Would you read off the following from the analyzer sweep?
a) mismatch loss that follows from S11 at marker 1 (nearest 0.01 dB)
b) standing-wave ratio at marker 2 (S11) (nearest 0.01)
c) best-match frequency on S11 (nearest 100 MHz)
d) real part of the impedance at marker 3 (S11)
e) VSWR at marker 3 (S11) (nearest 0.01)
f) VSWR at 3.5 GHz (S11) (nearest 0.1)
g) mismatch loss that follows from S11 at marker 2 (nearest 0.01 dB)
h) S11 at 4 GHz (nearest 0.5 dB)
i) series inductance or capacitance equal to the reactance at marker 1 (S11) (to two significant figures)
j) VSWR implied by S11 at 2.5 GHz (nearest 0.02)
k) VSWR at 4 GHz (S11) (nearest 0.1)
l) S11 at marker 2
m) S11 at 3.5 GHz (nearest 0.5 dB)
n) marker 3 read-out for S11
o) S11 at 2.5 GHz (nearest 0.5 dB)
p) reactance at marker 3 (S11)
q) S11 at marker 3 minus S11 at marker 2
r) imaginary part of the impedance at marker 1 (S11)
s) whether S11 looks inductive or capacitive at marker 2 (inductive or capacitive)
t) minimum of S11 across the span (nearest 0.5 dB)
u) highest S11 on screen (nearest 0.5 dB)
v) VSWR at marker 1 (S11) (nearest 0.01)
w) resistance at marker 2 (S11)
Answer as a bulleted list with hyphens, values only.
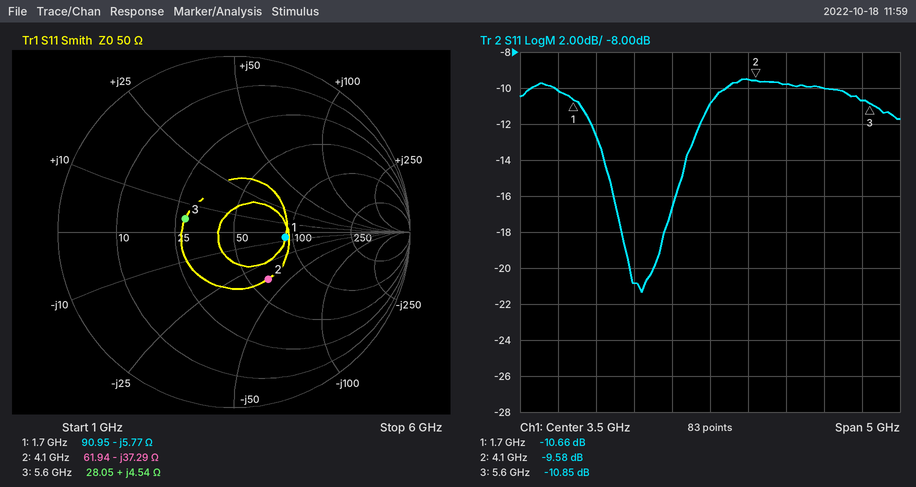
- 0.39 dB
- 1.99
- 2.6 GHz
- 28.05 Ω
- 1.80
- 1.8
- 0.51 dB
- -9.5 dB
- 16 pF
- 1.20
- 2.0
- -9.58 dB
- -11.0 dB
- -10.85 dB
- -21.0 dB
- +4.54 Ω
- -1.27 dB
- -5.77 Ω
- capacitive
- -21.5 dB
- -9.5 dB
- 1.83
- 61.94 Ω
